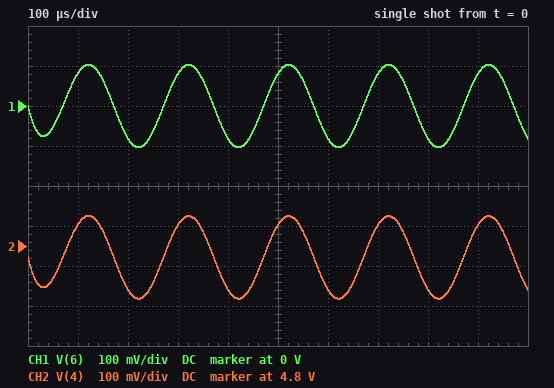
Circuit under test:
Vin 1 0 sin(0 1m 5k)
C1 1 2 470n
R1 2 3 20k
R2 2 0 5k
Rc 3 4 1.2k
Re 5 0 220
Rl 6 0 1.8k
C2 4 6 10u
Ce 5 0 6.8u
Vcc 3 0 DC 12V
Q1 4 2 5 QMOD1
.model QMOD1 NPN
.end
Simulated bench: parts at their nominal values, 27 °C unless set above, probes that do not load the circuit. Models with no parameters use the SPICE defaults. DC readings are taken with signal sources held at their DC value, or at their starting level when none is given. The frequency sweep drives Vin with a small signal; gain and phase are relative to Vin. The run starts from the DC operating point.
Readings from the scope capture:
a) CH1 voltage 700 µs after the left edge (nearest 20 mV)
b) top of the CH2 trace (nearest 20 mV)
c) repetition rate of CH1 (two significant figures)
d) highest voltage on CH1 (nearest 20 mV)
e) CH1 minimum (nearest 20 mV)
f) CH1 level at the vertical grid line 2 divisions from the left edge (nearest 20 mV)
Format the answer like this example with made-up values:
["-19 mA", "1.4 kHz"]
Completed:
["80 mV", "4.88 V", "5.0 kHz", "100 mV", "-100 mV", "-80 mV"]
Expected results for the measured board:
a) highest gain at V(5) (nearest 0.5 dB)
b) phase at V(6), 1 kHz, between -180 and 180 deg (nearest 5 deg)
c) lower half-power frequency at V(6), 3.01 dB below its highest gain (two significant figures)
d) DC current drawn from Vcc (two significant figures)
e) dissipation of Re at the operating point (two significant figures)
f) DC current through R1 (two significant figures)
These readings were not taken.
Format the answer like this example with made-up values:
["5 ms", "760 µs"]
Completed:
["-1.5 dB", "-100 deg", "6.4 kHz", "6.5 mA", "8.1 mW", "490 µA"]
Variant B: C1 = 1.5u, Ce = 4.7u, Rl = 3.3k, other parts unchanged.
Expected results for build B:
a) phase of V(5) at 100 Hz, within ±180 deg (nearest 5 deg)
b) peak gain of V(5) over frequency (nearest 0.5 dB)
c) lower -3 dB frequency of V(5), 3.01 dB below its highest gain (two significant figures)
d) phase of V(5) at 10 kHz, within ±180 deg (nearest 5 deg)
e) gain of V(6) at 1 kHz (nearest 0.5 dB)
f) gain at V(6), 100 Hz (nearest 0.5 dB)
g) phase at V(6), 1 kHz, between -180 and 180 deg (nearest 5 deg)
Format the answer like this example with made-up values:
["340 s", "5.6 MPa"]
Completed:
["15 deg", "-0.5 dB", "30 Hz", "-50 deg", "28.0 dB", "12.5 dB", "-105 deg"]
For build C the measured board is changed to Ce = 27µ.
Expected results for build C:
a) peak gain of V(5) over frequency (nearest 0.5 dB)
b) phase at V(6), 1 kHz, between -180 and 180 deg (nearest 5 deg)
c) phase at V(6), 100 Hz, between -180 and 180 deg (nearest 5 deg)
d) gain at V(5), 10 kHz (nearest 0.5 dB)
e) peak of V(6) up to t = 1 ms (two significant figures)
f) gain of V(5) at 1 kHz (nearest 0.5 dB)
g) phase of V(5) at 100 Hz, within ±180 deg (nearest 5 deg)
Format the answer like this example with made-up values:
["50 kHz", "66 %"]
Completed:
["-4.5 dB", "-110 deg", "-70 deg", "-17.5 dB", "160 mV", "-5.0 dB", "30 deg"]
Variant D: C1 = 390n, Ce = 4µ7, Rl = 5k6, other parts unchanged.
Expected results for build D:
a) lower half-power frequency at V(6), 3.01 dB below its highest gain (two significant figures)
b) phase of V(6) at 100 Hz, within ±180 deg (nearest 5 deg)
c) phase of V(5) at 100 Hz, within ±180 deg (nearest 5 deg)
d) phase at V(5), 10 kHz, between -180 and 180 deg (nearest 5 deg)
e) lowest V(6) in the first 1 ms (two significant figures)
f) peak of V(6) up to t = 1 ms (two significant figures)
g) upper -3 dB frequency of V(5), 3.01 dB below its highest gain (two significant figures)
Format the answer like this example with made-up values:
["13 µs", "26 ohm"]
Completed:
["9.1 kHz", "-100 deg", "45 deg", "-45 deg", "-110 mV", "110 mV", "9.3 kHz"]
